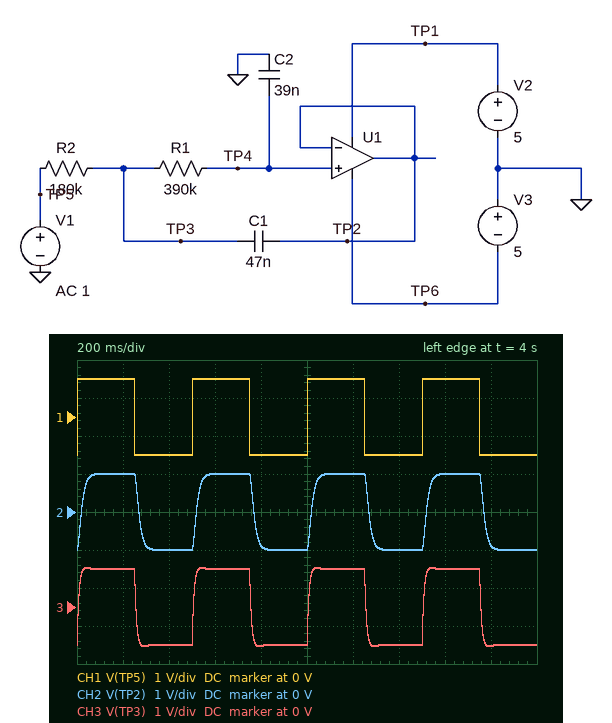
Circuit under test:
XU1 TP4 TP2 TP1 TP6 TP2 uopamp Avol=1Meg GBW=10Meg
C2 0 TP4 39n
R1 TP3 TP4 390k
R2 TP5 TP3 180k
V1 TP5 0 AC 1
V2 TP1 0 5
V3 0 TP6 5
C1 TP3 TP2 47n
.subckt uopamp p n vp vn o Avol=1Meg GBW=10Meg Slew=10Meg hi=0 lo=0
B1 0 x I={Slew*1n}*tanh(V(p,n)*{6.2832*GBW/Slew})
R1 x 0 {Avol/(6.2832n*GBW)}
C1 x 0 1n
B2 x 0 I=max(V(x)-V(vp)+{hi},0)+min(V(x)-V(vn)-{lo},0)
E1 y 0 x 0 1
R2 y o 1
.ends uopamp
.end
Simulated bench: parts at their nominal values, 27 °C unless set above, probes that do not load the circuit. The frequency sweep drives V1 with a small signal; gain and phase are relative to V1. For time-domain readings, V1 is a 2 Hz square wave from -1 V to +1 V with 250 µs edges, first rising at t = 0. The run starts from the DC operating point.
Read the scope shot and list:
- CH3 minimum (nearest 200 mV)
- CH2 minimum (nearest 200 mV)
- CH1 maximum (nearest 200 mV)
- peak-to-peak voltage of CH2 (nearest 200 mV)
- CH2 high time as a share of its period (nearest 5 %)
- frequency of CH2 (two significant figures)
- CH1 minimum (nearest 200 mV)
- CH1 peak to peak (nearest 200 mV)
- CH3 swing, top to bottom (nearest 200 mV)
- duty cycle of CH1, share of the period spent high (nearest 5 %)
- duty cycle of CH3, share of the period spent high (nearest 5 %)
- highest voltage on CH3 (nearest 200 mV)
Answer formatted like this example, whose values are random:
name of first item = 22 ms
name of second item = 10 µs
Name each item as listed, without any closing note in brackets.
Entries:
CH3 minimum = -1.0 V
CH2 minimum = -1.0 V
CH1 maximum = 1.0 V
peak-to-peak voltage of CH2 = 2.0 V
CH2 high time as a share of its period = 50 %
frequency of CH2 = 2.0 Hz
CH1 minimum = -1.0 V
CH1 peak to peak = 2.0 V
CH3 swing, top to bottom = 2.0 V
duty cycle of CH1, share of the period spent high = 50 %
duty cycle of CH3, share of the period spent high = 50 %
highest voltage on CH3 = 1.0 V
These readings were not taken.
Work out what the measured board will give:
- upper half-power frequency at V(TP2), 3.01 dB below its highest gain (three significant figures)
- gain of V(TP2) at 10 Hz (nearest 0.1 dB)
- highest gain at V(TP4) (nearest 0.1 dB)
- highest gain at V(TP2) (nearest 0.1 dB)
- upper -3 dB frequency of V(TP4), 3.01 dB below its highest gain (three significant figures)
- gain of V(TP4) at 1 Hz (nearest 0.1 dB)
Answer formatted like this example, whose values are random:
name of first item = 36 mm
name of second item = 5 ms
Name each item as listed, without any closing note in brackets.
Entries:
upper half-power frequency at V(TP2), 3.01 dB below its highest gain = 9.29 Hz
gain of V(TP2) at 10 Hz = -3.4 dB
highest gain at V(TP4) = 0 dB
highest gain at V(TP2) = 0 dB
upper -3 dB frequency of V(TP4), 3.01 dB below its highest gain = 9.29 Hz
gain of V(TP4) at 1 Hz = 0 dB
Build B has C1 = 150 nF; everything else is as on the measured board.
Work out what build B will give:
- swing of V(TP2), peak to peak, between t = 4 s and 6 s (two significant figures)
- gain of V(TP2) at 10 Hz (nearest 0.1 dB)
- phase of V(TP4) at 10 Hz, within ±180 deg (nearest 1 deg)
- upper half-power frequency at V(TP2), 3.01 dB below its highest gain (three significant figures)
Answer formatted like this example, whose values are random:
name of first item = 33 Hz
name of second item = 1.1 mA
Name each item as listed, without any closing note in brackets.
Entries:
swing of V(TP2), peak to peak, between t = 4 s and 6 s = 2.5 V
gain of V(TP2) at 10 Hz = -3.7 dB
phase of V(TP4) at 10 Hz, within ±180 deg = -114 deg
upper half-power frequency at V(TP2), 3.01 dB below its highest gain = 9.01 Hz
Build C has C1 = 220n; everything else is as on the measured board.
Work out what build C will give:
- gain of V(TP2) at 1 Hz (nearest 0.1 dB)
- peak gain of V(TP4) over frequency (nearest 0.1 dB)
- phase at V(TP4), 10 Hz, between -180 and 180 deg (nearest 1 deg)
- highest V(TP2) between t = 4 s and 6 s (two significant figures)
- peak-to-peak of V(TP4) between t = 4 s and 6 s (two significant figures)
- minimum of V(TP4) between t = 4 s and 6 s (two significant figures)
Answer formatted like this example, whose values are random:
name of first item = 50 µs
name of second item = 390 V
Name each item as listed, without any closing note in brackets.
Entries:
gain of V(TP2) at 1 Hz = 0.1 dB
peak gain of V(TP4) over frequency = 1.9 dB
phase at V(TP4), 10 Hz, between -180 and 180 deg = -135 deg
highest V(TP2) between t = 4 s and 6 s = 1.4 V
peak-to-peak of V(TP4) between t = 4 s and 6 s = 2.8 V
minimum of V(TP4) between t = 4 s and 6 s = -1.4 V
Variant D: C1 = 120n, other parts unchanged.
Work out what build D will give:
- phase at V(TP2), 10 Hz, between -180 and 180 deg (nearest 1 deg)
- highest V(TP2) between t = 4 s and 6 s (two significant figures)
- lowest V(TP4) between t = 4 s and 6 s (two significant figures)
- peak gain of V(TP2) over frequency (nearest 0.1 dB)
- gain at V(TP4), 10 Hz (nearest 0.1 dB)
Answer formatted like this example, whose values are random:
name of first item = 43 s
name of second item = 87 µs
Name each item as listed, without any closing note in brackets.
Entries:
phase at V(TP2), 10 Hz, between -180 and 180 deg = -102 deg
highest V(TP2) between t = 4 s and 6 s = 1.2 V
lowest V(TP4) between t = 4 s and 6 s = -1.2 V
peak gain of V(TP2) over frequency = 0.3 dB
gain at V(TP4), 10 Hz = -3.1 dB
